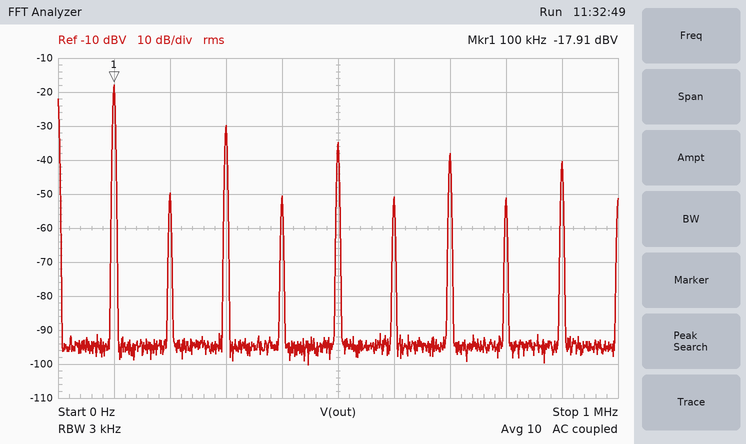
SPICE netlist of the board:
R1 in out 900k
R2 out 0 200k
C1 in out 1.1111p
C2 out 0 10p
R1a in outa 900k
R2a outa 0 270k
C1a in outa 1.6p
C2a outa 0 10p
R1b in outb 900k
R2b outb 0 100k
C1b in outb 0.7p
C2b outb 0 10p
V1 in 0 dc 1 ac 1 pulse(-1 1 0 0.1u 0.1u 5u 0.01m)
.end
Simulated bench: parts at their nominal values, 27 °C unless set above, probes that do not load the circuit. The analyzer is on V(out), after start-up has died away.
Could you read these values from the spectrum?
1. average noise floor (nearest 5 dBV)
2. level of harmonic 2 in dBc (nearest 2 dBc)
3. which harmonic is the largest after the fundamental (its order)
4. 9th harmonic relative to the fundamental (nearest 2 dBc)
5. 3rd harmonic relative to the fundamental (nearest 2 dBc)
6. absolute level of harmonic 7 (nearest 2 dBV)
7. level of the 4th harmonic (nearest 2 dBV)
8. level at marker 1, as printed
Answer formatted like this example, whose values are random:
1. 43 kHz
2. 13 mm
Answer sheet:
1. -95 dBV
2. -32 dBc
3. 3
4. -22 dBc
5. -12 dBc
6. -38 dBV
7. -50 dBV
8. -17.91 dBV
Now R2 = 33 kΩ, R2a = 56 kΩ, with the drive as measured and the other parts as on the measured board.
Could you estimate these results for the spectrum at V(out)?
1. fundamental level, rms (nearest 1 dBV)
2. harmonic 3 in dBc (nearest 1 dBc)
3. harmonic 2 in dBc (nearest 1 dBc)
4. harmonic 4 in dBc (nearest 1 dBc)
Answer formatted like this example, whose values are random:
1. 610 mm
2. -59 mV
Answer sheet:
1. -29 dBV
2. -6 dBc
3. -28 dBc
4. -25 dBc
